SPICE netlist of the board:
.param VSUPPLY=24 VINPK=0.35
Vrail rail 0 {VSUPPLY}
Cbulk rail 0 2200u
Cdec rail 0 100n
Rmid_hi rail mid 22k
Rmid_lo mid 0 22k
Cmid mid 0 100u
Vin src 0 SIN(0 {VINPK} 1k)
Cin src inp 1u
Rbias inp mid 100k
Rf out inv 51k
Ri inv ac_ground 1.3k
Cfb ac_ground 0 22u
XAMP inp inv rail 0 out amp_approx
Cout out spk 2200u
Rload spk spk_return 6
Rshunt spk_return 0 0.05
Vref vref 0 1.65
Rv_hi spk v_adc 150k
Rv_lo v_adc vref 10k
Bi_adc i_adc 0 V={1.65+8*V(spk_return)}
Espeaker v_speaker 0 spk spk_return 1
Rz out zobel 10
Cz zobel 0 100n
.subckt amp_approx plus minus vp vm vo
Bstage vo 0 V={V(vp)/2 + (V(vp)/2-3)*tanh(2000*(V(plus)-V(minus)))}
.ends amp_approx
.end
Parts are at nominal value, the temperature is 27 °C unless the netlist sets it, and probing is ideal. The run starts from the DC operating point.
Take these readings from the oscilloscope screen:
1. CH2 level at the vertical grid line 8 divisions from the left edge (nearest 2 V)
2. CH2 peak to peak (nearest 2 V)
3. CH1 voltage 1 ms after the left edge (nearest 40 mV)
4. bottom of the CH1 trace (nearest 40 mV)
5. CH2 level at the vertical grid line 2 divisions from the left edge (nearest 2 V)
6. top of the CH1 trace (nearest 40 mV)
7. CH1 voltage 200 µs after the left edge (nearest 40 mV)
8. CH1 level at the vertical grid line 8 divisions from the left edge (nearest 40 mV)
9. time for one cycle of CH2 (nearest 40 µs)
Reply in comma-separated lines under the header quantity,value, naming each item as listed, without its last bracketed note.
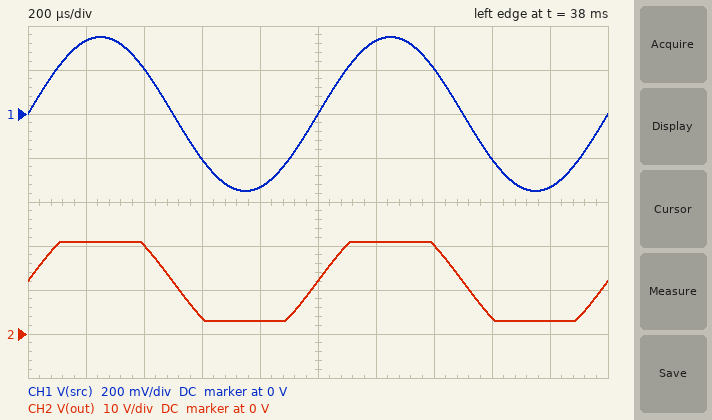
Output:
quantity,value
CH2 level at the vertical grid line 8 divisions from the left edge,4 V
CH2 peak to peak,18 V
CH1 voltage 1 ms after the left edge,0 V
bottom of the CH1 trace,-360 mV
CH2 level at the vertical grid line 2 divisions from the left edge,20 V
top of the CH1 trace,360 mV
CH1 voltage 200 µs after the left edge,320 mV
CH1 level at the vertical grid line 8 divisions from the left edge,-200 mV
time for one cycle of CH2,1.00 ms
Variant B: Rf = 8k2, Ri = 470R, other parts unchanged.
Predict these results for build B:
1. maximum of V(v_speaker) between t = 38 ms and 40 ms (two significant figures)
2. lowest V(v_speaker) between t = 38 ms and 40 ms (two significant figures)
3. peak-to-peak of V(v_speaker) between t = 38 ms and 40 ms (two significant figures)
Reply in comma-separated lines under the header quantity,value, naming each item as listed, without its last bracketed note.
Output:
quantity,value
maximum of V(v_speaker) between t = 38 ms and 40 ms,6.4 V
lowest V(v_speaker) between t = 38 ms and 40 ms,-6.4 V
peak-to-peak of V(v_speaker) between t = 38 ms and 40 ms,13 V
